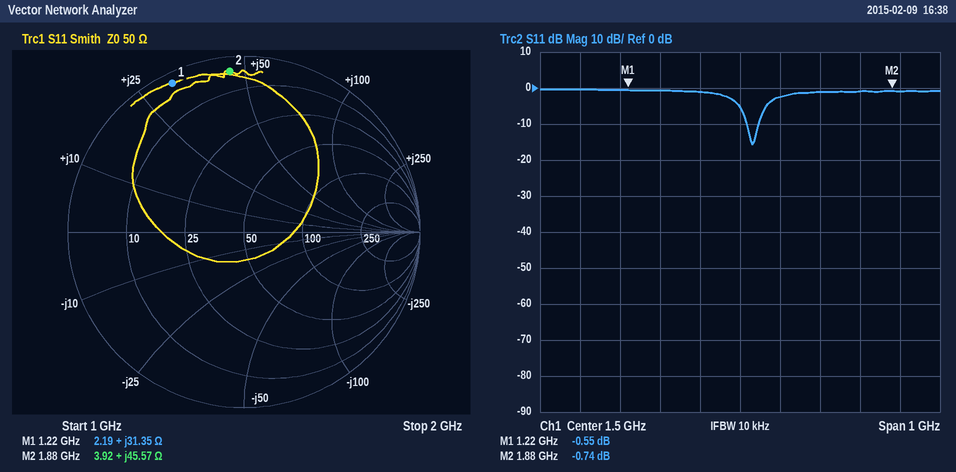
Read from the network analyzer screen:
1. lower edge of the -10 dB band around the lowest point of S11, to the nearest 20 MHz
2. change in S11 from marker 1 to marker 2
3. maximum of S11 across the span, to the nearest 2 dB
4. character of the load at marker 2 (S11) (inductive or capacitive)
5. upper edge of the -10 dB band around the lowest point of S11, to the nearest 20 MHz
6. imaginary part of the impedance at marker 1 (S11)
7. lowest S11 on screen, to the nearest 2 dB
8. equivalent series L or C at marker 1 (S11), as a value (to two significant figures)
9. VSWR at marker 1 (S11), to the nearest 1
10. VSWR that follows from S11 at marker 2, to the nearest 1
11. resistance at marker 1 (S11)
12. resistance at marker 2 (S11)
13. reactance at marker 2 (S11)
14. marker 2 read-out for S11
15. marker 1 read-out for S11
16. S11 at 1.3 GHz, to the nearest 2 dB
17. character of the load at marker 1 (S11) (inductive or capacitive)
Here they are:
1.52 GHz
-0.19 dB
0 dB
inductive
1.54 GHz
+31.35 Ω
-16 dB
4.1 nH
32
23
2.19 Ω
3.92 Ω
+45.57 Ω
-0.74 dB
-0.55 dB
0 dB
inductive
